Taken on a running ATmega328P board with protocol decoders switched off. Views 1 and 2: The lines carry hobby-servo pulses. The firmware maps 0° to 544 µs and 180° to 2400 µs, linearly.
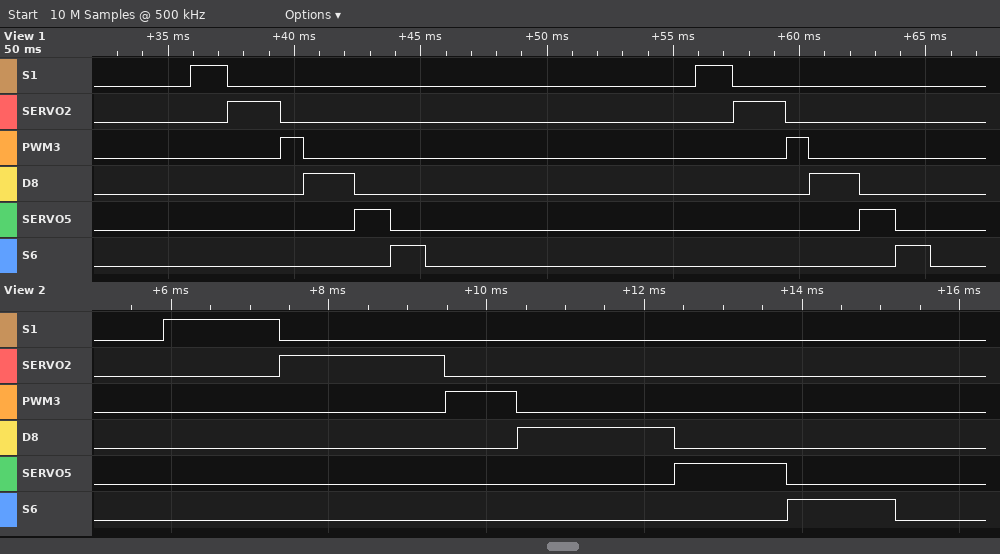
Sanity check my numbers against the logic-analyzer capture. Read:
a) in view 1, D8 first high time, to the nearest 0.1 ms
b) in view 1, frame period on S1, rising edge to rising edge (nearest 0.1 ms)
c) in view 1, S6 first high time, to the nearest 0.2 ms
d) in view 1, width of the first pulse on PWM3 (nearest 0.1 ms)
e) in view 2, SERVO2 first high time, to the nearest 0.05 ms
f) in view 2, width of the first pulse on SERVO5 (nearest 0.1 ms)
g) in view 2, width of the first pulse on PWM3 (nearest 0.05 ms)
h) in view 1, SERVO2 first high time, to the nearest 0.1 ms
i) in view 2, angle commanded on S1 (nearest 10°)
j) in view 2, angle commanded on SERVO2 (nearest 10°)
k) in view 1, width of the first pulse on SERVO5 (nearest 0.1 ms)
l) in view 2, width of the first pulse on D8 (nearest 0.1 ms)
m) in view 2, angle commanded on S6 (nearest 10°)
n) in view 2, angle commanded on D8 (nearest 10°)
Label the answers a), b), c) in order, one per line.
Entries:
a) 2.0 ms
b) 20.0 ms
c) 1.4 ms
d) 0.9 ms
e) 2.10 ms
f) 1.4 ms
g) 0.90 ms
h) 2.1 ms
i) 90°
j) 150°
k) 1.4 ms
l) 2.0 ms
m) 80°
n) 140°
